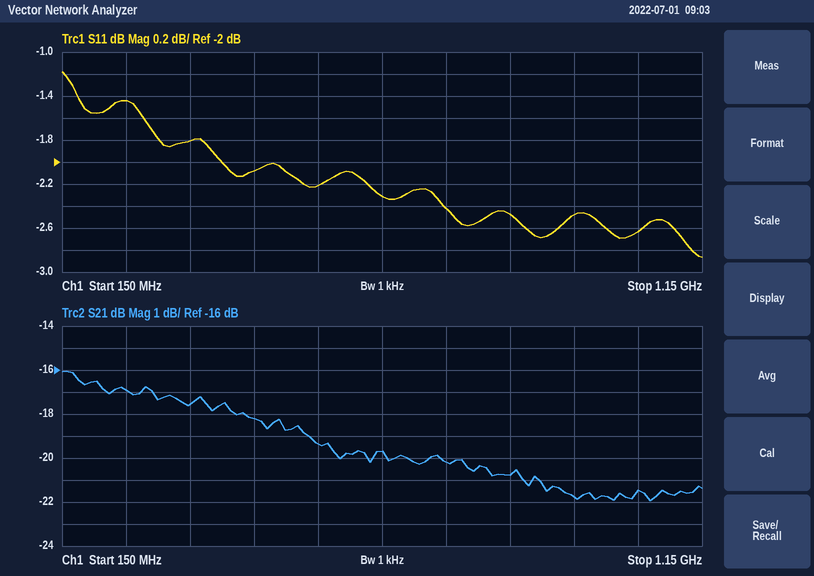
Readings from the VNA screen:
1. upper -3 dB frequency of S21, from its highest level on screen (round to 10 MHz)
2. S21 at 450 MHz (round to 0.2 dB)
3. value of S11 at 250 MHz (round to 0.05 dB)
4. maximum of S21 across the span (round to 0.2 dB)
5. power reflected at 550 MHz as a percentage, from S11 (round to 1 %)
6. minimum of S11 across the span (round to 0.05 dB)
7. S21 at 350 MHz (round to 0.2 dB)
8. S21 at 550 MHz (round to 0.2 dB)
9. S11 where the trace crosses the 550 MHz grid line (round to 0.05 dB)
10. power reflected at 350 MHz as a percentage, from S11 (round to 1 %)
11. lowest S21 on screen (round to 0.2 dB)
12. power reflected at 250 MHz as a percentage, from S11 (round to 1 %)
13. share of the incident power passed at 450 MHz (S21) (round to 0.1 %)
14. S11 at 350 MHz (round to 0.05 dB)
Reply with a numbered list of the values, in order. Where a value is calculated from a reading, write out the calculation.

1. 540 MHz
2. -18.2 dB
3. -1.45 dB
4. -16.0 dB
5. 10^(-2.2/10) ≈ 60 %
6. -2.85 dB
7. -17.6 dB
8. -19.4 dB
9. -2.20 dB
10. 10^(-1.8/10) ≈ 66 %
11. -22.0 dB
12. 10^(-1.45/10) ≈ 72 %
13. 10^(-18.2/10) ≈ 1.5 %
14. -1.80 dB
